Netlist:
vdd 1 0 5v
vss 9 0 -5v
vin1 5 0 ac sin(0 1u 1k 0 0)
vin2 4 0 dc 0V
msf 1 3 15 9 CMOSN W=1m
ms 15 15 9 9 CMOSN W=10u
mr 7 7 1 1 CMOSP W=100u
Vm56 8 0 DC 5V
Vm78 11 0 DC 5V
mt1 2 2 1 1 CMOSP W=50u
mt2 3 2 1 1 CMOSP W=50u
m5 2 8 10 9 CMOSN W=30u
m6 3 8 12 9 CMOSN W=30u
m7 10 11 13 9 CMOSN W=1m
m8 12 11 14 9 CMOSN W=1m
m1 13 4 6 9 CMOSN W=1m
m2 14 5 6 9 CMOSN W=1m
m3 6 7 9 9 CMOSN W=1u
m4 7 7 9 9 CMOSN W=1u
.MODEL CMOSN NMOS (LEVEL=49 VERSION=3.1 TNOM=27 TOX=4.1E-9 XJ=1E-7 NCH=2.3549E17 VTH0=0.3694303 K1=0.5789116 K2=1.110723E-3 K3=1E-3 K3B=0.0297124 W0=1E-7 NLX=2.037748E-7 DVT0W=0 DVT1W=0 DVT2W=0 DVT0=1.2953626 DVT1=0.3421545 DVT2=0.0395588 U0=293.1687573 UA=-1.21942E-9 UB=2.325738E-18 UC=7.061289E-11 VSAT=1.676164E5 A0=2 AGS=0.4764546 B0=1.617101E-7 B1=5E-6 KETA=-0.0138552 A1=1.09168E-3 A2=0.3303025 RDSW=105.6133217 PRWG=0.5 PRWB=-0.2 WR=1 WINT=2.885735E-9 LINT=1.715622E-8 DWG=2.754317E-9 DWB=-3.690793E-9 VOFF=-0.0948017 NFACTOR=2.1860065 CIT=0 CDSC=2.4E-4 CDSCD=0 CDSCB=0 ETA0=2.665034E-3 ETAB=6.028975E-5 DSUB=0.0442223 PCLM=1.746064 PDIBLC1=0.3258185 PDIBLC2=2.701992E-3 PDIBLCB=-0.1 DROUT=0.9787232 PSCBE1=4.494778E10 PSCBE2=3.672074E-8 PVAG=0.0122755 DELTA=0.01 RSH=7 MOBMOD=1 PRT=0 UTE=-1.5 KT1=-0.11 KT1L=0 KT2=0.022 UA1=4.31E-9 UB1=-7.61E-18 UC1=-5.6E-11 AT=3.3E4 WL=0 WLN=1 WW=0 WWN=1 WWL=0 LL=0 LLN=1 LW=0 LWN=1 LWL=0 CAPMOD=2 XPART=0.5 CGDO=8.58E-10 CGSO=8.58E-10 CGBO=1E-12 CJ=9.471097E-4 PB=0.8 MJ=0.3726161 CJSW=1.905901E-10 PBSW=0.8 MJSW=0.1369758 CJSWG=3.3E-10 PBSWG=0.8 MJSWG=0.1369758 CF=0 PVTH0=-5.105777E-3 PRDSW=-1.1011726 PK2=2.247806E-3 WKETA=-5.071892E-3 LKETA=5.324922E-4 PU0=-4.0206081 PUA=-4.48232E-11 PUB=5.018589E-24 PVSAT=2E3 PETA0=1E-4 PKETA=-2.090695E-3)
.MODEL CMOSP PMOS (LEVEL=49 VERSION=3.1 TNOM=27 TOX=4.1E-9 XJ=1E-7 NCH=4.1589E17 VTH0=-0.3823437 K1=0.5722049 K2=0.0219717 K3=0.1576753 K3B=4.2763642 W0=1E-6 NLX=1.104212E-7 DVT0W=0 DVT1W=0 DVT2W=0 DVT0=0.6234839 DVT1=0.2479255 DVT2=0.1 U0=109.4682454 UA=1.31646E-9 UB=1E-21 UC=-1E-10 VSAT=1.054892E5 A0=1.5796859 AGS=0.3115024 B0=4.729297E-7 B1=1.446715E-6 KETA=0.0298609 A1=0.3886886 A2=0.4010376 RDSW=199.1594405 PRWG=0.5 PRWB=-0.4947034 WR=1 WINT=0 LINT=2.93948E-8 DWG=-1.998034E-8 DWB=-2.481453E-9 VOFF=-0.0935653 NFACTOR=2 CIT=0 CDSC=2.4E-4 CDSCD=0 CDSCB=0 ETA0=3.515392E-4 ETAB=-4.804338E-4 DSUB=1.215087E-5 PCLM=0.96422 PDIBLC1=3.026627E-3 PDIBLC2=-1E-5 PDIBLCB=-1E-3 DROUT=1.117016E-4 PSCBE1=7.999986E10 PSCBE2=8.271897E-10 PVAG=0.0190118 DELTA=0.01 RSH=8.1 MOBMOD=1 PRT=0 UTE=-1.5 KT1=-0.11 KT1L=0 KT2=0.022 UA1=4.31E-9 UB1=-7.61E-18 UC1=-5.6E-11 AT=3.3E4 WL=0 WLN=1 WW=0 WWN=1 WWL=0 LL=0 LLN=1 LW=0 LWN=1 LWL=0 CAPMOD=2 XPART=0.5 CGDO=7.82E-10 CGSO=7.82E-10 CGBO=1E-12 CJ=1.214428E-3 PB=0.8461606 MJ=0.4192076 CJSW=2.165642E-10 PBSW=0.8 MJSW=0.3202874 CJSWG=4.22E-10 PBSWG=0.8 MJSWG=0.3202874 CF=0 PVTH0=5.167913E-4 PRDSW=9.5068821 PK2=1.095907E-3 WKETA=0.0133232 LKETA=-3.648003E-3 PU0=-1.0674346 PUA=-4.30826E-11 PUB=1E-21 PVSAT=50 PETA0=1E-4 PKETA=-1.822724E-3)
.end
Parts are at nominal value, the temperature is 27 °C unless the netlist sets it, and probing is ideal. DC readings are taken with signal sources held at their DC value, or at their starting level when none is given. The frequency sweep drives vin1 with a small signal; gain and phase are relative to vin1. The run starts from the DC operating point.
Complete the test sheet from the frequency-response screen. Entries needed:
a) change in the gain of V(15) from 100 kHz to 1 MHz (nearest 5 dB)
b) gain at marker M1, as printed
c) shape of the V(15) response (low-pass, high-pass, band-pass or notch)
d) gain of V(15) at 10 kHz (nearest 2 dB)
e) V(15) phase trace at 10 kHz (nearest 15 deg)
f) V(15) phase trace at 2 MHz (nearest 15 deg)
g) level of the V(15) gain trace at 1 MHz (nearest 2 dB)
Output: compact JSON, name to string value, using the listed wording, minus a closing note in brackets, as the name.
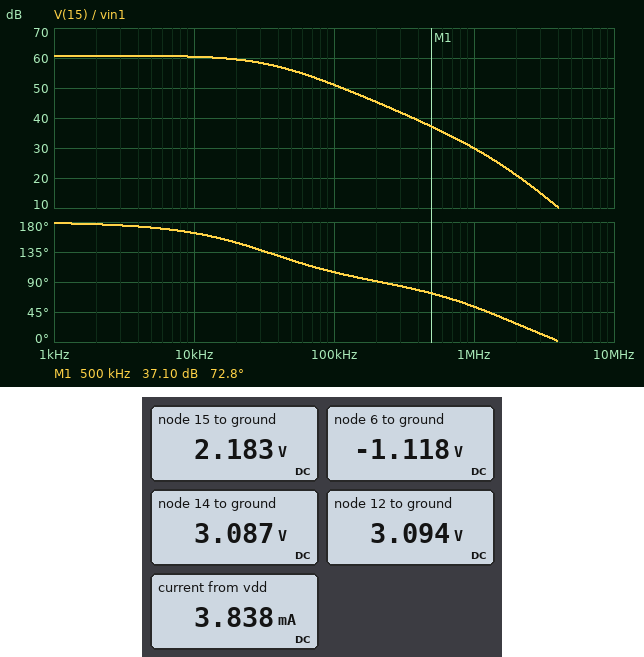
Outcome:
{"change in the gain of V(15) from 100 kHz to 1 MHz": "-20 dB", "gain at marker M1, as printed": "37.10 dB", "shape of the V(15) response": "low-pass", "gain of V(15) at 10 kHz": "60 dB", "V(15) phase trace at 10 kHz": "165 deg", "V(15) phase trace at 2 MHz": "30 deg", "level of the V(15) gain trace at 1 MHz": "30 dB"}
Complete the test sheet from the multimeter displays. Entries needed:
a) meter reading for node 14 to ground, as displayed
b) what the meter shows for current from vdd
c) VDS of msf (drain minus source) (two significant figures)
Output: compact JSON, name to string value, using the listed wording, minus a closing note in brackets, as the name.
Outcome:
{"meter reading for node 14 to ground, as displayed": "3.087 V", "what the meter shows for current from vdd": "3.838 mA", "VDS of msf (drain minus source)": "2.8 V"}
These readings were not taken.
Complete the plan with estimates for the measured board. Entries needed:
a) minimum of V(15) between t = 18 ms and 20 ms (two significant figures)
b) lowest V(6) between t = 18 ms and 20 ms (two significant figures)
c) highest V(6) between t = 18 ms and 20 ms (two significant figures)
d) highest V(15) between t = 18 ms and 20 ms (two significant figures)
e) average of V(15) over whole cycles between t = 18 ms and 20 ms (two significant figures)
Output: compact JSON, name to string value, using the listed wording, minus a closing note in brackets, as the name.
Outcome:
{"minimum of V(15) between t = 18 ms and 20 ms": "2.2 V", "lowest V(6) between t = 18 ms and 20 ms": "-1.1 V", "highest V(6) between t = 18 ms and 20 ms": "-1.1 V", "highest V(15) between t = 18 ms and 20 ms": "2.2 V", "average of V(15) over whole cycles between t = 18 ms and 20 ms": "2.2 V"}
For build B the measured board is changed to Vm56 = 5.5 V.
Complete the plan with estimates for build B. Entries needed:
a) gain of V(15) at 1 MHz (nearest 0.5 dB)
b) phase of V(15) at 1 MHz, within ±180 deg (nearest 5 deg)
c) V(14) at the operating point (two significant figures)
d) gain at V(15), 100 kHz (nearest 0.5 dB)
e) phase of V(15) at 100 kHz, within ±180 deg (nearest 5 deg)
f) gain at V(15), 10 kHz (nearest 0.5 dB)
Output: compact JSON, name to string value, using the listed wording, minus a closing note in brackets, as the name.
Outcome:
{"gain of V(15) at 1 MHz": "32.0 dB", "phase of V(15) at 1 MHz, within ±180 deg": "80 deg", "V(14) at the operating point": "3.4 V", "gain at V(15), 100 kHz": "51.5 dB", "phase of V(15) at 100 kHz, within ±180 deg": "110 deg", "gain at V(15), 10 kHz": "60.5 dB"}
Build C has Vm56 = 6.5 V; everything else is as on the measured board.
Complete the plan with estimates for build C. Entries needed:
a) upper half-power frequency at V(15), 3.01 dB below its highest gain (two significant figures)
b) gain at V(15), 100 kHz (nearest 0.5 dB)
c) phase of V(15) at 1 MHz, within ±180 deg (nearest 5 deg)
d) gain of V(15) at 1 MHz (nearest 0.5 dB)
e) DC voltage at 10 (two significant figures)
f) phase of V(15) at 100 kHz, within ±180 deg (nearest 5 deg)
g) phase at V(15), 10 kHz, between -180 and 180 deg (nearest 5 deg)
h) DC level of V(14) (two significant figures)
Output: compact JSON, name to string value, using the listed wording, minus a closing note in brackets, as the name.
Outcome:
{"upper half-power frequency at V(15), 3.01 dB below its highest gain": "26 kHz", "gain at V(15), 100 kHz": "49.0 dB", "phase of V(15) at 1 MHz, within ±180 deg": "80 deg", "gain of V(15) at 1 MHz": "29.0 dB", "DC voltage at 10": "4.0 V", "phase of V(15) at 100 kHz, within ±180 deg": "105 deg", "phase at V(15), 10 kHz, between -180 and 180 deg": "160 deg", "DC level of V(14)": "3.4 V"}
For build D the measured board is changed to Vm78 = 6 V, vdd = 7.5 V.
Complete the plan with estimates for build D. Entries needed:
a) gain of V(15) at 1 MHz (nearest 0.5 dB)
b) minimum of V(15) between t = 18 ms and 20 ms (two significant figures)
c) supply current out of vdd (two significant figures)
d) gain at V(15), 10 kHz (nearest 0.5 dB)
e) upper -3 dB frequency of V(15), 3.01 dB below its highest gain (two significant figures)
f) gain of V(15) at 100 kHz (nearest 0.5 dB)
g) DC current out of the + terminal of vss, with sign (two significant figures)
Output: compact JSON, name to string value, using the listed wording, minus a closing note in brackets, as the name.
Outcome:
{"gain of V(15) at 1 MHz": "28.5 dB", "minimum of V(15) between t = 18 ms and 20 ms": "4.5 V", "supply current out of vdd": "3.9 mA", "gain at V(15), 10 kHz": "60.0 dB", "upper -3 dB frequency of V(15), 3.01 dB below its highest gain": "32 kHz", "gain of V(15) at 100 kHz": "50.0 dB", "DC current out of the + terminal of vss, with sign": "-3.9 mA"}
